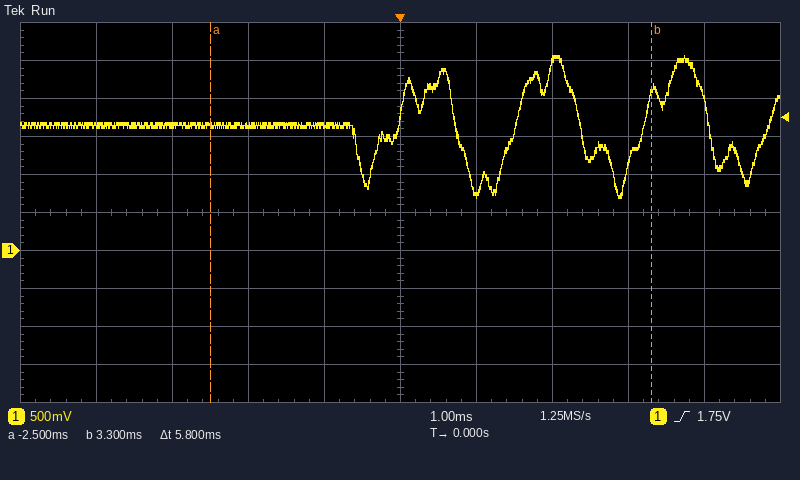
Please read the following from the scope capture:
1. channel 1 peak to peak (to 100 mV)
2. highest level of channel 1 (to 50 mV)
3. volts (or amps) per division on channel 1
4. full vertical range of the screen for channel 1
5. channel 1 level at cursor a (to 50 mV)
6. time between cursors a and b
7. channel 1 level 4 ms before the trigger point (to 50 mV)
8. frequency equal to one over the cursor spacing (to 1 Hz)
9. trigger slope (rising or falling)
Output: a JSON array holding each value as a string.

["1.90 V", "2.55 V", "500 mV", "5 V", "1.65 V", "5.8 ms", "1.65 V", "172 Hz", "rising"]
